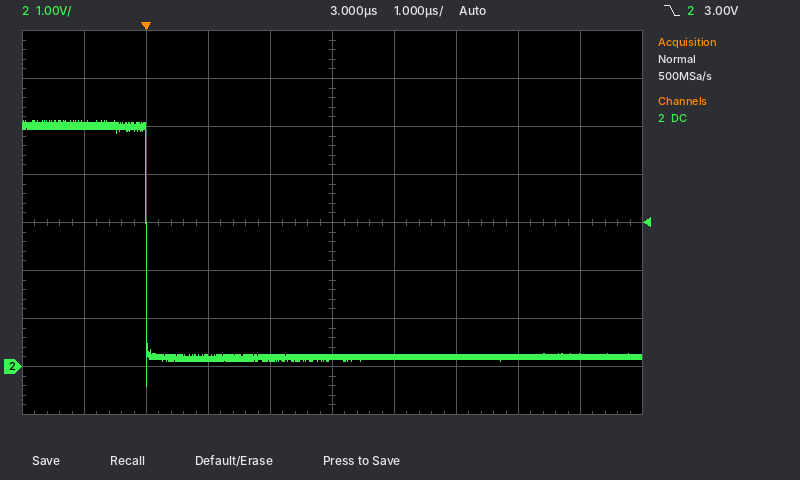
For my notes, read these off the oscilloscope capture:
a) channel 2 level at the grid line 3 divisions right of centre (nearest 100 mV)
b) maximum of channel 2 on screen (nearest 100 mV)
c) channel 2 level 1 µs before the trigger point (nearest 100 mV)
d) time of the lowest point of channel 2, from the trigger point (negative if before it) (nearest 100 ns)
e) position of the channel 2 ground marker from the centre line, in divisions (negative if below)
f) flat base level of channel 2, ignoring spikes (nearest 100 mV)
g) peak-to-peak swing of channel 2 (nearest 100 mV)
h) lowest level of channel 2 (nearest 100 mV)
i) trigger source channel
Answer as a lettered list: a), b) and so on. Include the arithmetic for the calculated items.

a) 200 mV
b) 5.1 V
c) 5.0 V
d) 0.0 µs
e) -3.0 div
f) 200 mV
g) 5.1 V − (-400 mV) = 5.5 V
h) -400 mV
i) channel 2
